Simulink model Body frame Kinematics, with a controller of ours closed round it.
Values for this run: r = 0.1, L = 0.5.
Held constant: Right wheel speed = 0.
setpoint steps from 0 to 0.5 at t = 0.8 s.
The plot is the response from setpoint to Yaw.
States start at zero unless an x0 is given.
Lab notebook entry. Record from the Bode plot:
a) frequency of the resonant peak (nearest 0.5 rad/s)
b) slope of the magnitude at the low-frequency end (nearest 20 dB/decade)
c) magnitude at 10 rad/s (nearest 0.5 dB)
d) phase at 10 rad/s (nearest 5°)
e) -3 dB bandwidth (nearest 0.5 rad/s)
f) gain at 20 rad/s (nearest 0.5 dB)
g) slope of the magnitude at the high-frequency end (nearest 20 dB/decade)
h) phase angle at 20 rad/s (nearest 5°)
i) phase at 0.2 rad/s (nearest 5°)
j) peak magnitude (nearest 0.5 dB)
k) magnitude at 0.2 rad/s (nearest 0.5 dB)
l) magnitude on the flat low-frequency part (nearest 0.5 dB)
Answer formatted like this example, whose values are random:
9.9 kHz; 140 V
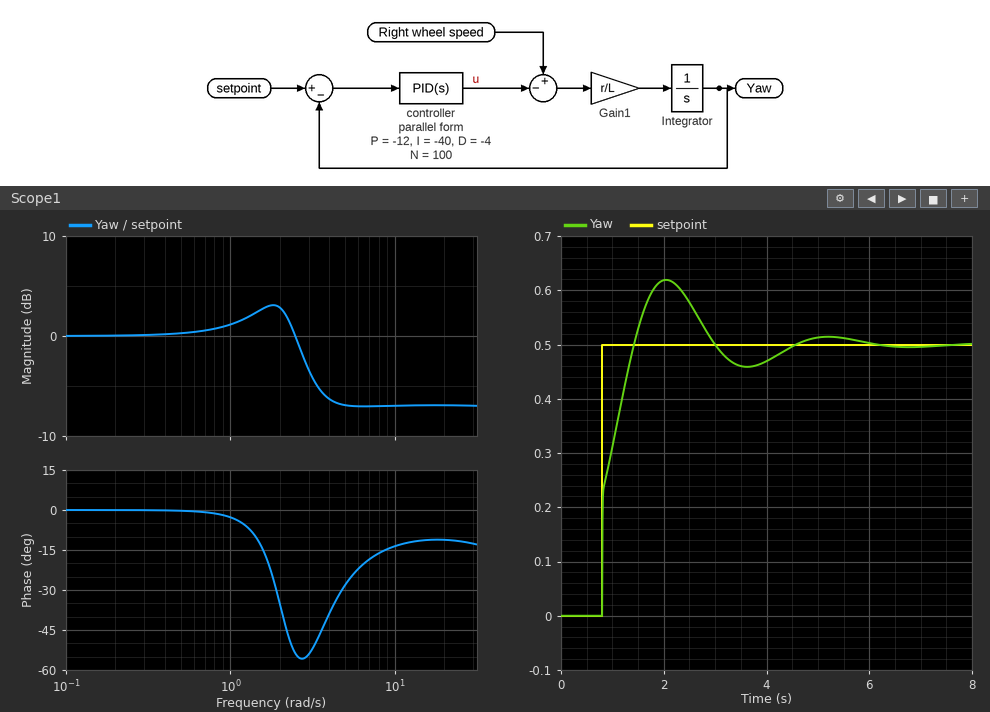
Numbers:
2.0 rad/s; 0 dB/decade; -7.0 dB; -15°; 3.0 rad/s; -7.0 dB; 0 dB/decade; -10°; 0°; 3.0 dB; 0.0 dB; 0.0 dB
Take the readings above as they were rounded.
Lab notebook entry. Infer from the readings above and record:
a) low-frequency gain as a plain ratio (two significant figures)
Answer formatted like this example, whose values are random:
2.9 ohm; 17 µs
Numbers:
1.0
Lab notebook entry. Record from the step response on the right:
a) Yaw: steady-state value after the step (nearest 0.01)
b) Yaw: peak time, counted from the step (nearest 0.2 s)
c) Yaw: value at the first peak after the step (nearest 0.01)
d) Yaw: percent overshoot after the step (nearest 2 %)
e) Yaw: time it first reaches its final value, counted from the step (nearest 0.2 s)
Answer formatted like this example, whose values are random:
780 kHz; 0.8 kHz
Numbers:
0.50; 1.2 s; 0.62; 24 %; 0.6 s
